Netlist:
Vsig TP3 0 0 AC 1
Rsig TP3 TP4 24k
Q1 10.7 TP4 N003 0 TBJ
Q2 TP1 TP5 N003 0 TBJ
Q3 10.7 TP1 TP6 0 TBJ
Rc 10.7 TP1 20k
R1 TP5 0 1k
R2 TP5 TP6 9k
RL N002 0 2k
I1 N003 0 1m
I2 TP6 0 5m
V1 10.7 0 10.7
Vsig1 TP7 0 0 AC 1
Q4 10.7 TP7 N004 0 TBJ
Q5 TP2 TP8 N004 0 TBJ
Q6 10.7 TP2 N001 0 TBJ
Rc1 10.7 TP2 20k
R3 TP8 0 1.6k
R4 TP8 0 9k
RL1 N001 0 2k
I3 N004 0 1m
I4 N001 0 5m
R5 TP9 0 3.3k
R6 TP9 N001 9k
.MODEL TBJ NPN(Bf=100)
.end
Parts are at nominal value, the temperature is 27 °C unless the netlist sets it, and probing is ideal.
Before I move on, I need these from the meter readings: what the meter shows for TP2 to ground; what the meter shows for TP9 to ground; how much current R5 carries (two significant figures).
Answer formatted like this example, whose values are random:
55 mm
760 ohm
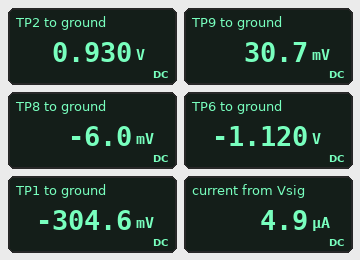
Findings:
0.930 V
30.7 mV
9.3 µA
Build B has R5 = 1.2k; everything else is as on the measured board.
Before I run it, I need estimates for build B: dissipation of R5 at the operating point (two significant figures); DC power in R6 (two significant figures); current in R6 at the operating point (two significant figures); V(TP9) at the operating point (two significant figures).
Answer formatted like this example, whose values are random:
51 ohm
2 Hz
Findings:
150 nW
1.1 µW
11 µA
13 mV
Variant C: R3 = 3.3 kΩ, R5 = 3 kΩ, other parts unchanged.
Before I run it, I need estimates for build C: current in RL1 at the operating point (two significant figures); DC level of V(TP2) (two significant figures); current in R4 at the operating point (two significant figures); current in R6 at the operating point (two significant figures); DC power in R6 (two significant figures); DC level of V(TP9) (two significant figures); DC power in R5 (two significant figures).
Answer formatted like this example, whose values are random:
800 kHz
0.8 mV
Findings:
370 µA
1.6 V
1.1 µA
62 µA
35 µW
190 mV
12 µW
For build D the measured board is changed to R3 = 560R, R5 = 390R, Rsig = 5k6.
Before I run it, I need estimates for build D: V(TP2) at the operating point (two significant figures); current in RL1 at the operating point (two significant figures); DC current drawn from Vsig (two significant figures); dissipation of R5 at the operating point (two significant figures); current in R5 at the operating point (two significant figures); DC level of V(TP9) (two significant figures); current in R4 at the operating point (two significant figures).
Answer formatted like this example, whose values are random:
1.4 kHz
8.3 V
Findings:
340 mV
240 µA
5.3 µA
990 nW
50 µA
-20 mV
280 nA
